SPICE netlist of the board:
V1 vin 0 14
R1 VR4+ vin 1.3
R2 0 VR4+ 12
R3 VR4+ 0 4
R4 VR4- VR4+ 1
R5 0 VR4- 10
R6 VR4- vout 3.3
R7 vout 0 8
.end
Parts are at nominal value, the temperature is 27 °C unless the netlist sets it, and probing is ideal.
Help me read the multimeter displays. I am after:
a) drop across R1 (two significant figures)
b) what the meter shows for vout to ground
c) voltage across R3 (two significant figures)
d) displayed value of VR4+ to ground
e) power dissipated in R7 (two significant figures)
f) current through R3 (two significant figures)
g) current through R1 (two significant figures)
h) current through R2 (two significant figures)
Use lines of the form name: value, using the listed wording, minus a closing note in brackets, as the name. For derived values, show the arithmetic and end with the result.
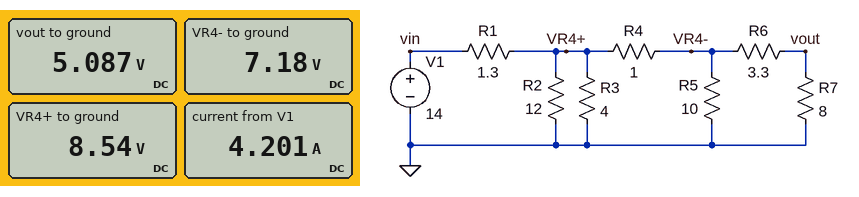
drop across R1: 14 V - 8.54 V = 5.5 V
what the meter shows for vout to ground: 5.087 V
voltage across R3: 8.54 V = 8.5 V
displayed value of VR4+ to ground: 8.54 V
power dissipated in R7: (5.087 V)^2 / 8 Ω = 3.2 W
current through R3: (8.54 V) / 4 Ω = 2.1 A
current through R1: (14 V - 8.54 V) / 1.3 Ω = 4.2 A
current through R2: (8.54 V) / 12 Ω = 710 mA
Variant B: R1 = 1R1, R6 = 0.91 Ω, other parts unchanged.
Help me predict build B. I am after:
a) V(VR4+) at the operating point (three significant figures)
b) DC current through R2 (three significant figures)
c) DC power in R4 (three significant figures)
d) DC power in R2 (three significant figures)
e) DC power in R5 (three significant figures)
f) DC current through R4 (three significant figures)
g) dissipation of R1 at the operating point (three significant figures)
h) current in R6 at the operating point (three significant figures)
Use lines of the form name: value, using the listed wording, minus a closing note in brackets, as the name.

V(VR4+) at the operating point: 8.98 V
DC current through R2: 748 mA
DC power in R4: 2.47 W
DC power in R2: 6.72 W
DC power in R5: 5.49 W
DC current through R4: 1.57 A
dissipation of R1 at the operating point: 22.9 W
current in R6 at the operating point: 831 mA
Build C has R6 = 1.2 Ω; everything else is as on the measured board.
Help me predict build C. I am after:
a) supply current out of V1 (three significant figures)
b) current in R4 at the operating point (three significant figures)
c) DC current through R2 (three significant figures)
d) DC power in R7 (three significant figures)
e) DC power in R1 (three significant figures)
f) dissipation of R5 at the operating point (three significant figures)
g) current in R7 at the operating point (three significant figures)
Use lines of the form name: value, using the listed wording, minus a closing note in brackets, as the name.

supply current out of V1: 4.27 A
current in R4 at the operating point: 1.46 A
DC current through R2: 704 mA
DC power in R7: 4.61 W
DC power in R1: 23.7 W
dissipation of R5 at the operating point: 4.88 W
current in R7 at the operating point: 759 mA
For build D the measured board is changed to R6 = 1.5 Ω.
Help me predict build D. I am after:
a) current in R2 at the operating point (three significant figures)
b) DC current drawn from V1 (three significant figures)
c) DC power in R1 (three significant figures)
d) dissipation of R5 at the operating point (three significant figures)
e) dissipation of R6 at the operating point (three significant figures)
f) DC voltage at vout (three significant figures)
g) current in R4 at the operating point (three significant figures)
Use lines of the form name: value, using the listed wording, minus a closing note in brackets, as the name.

current in R2 at the operating point: 705 mA
DC current drawn from V1: 4.26 A
DC power in R1: 23.6 W
dissipation of R5 at the operating point: 4.93 W
dissipation of R6 at the operating point: 819 mW
DC voltage at vout: 5.91 V
current in R4 at the operating point: 1.44 A
